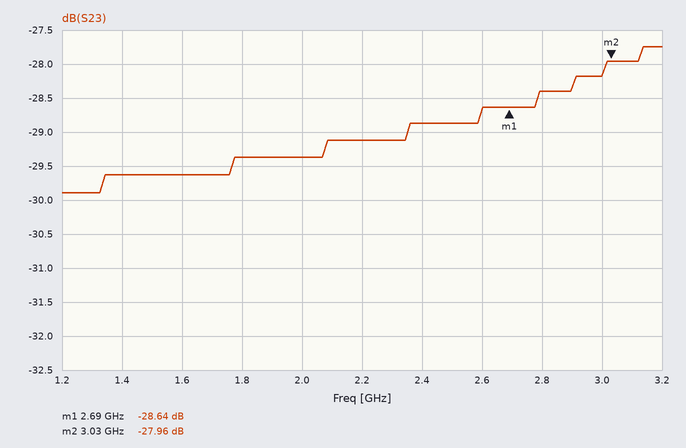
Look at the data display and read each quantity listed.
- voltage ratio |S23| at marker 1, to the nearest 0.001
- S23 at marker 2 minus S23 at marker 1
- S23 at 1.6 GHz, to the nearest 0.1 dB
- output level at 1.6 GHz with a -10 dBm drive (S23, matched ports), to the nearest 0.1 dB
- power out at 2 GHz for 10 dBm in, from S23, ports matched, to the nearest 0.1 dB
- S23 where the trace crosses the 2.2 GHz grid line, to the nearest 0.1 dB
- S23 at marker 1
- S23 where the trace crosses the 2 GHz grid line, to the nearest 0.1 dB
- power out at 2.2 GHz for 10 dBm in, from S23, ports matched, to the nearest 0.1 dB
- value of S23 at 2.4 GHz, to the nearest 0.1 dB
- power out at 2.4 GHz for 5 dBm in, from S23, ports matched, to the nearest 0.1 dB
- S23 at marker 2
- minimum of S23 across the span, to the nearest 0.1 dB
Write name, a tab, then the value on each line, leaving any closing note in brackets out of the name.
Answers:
voltage ratio |S23| at marker 1, to the nearest 0.001	0.037
S23 at marker 2 minus S23 at marker 1	0.68 dB
S23 at 1.6 GHz, to the nearest 0.1 dB	-29.6 dB
output level at 1.6 GHz with a -10 dBm drive (S23, matched ports), to the nearest 0.1 dB	-39.6 dBm
power out at 2 GHz for 10 dBm in, from S23, ports matched, to the nearest 0.1 dB	-19.4 dBm
S23 where the trace crosses the 2.2 GHz grid line, to the nearest 0.1 dB	-29.1 dB
S23 at marker 1	-28.64 dB
S23 where the trace crosses the 2 GHz grid line, to the nearest 0.1 dB	-29.4 dB
power out at 2.2 GHz for 10 dBm in, from S23, ports matched, to the nearest 0.1 dB	-19.1 dBm
value of S23 at 2.4 GHz, to the nearest 0.1 dB	-28.9 dB
power out at 2.4 GHz for 5 dBm in, from S23, ports matched, to the nearest 0.1 dB	-23.9 dBm
S23 at marker 2	-27.96 dB
minimum of S23 across the span, to the nearest 0.1 dB	-29.9 dB
